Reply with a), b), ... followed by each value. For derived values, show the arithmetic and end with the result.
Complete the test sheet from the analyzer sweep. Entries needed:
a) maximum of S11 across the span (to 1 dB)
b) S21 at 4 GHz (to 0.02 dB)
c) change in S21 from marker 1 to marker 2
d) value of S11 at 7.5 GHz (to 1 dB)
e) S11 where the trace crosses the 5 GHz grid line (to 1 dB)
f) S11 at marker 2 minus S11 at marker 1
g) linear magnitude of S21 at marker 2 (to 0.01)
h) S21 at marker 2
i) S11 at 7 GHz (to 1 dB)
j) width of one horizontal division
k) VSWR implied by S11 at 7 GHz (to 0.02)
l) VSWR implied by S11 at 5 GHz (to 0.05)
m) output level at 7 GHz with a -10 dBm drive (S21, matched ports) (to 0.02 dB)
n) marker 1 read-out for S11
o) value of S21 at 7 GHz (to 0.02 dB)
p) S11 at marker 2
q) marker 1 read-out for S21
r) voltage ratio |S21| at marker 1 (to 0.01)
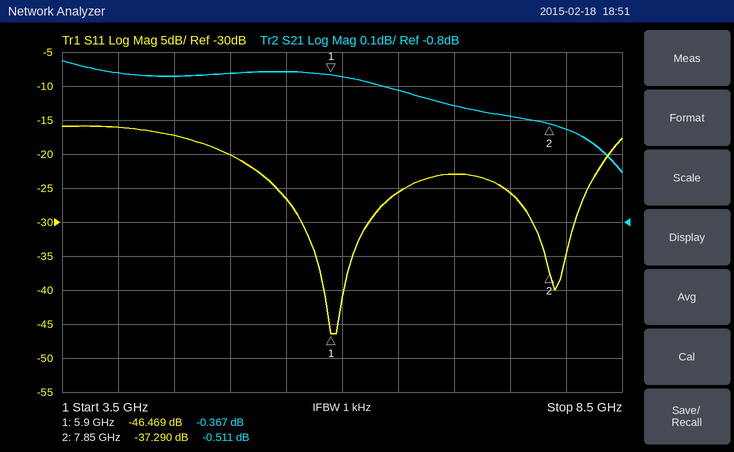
a) -16 dB
b) -0.36 dB
c) -0.511 − (-0.367) = -0.144 dB
d) -26 dB
e) -20 dB
f) -37.29 − (-46.469) = 9.179 dB
g) 10^(-0.511/20) ≈ 0.94
h) -0.511 dB
i) -23 dB
j) 500 MHz
k) |Γ| = 10^(-23/20) = 0.0708; VSWR = (1 + 0.0708)/(1 − 0.0708) ≈ 1.15, so 1.16 to the nearest 0.02
l) |Γ| = 10^(-20/20) = 0.1000; VSWR = (1 + 0.1000)/(1 − 0.1000) ≈ 1.22, so 1.20 to the nearest 0.05
m) -10 dBm + (-0.46 dB) = -10.46 dBm
n) -46.469 dB
o) -0.46 dB
p) -37.290 dB
q) -0.367 dB
r) 10^(-0.367/20) ≈ 0.96
